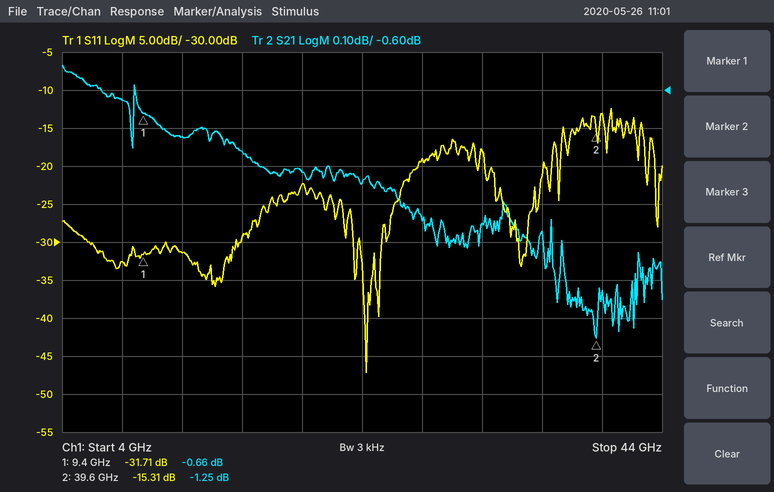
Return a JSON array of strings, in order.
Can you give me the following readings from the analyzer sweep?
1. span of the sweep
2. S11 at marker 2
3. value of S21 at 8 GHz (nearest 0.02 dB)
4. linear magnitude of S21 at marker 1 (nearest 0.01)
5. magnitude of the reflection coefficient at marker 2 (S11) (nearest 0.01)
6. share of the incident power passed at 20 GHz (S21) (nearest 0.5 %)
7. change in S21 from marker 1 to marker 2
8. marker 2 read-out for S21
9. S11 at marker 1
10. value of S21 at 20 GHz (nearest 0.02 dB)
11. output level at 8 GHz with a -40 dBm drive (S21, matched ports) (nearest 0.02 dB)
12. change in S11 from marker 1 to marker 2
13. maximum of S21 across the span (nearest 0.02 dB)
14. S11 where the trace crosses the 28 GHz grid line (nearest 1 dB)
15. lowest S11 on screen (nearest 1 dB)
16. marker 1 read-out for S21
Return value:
["40 GHz", "-15.31 dB", "-0.62 dB", "0.93", "0.17", "83.0 %", "-0.59 dB", "-1.25 dB", "-31.71 dB", "-0.82 dB", "-40.62 dBm", "16.40 dB", "-0.54 dB", "-19 dB", "-47 dB", "-0.66 dB"]
